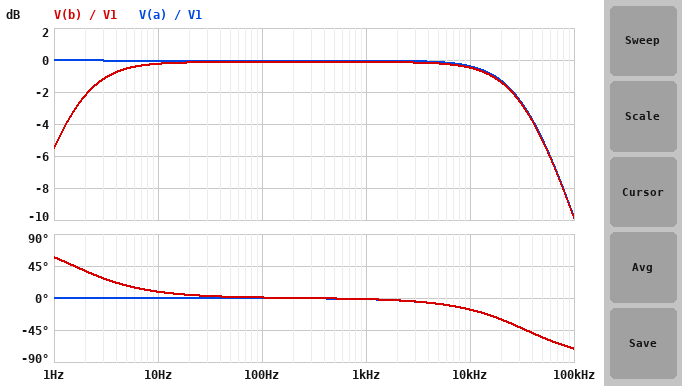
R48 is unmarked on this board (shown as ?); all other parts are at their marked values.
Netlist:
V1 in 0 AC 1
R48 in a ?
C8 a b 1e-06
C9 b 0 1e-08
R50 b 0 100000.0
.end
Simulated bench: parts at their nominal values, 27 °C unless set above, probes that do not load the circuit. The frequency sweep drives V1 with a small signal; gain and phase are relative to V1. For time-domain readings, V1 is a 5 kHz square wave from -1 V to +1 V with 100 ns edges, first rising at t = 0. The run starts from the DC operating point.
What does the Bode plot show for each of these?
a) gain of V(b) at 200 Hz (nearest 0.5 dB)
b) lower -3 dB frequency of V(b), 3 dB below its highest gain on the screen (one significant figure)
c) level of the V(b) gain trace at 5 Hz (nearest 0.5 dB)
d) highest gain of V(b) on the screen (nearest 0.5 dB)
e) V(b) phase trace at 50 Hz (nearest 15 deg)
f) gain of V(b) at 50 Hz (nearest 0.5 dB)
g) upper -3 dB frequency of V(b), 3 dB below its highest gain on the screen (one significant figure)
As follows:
0 dB
2 Hz
-0.5 dB
0 dB
0 deg
0 dB
30 kHz
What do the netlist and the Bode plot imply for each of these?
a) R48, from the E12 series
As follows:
470 Ω
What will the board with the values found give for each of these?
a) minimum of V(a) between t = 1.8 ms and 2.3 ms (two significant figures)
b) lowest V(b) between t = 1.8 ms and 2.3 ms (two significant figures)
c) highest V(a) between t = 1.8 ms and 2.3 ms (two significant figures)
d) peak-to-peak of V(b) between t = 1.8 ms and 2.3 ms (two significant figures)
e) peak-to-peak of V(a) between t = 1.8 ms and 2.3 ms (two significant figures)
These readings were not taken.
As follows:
-1.0 V
-21 mV
990 mV
2.0 V
2.0 V
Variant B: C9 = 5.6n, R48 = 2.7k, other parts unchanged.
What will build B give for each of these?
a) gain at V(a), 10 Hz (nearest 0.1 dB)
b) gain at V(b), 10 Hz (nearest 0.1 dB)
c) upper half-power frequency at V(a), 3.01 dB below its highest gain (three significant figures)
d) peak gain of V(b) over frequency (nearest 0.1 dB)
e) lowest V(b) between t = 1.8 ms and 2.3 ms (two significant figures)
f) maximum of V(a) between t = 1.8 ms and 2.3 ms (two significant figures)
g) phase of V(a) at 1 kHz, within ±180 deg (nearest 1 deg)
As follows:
-0.2 dB
-0.4 dB
10.3 kHz
-0.3 dB
-18 mV
950 mV
-5 deg
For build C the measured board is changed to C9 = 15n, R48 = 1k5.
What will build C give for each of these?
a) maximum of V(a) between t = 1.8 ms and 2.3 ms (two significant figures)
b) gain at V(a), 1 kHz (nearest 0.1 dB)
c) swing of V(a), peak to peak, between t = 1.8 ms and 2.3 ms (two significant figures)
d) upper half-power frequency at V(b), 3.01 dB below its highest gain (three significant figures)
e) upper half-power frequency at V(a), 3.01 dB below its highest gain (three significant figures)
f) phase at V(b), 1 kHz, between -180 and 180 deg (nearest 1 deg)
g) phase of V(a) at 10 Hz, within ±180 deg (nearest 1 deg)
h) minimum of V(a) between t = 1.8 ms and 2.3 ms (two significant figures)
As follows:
950 mV
-0.2 dB
1.9 V
7.29 kHz
7.07 kHz
-8 deg
0 deg
-980 mV
